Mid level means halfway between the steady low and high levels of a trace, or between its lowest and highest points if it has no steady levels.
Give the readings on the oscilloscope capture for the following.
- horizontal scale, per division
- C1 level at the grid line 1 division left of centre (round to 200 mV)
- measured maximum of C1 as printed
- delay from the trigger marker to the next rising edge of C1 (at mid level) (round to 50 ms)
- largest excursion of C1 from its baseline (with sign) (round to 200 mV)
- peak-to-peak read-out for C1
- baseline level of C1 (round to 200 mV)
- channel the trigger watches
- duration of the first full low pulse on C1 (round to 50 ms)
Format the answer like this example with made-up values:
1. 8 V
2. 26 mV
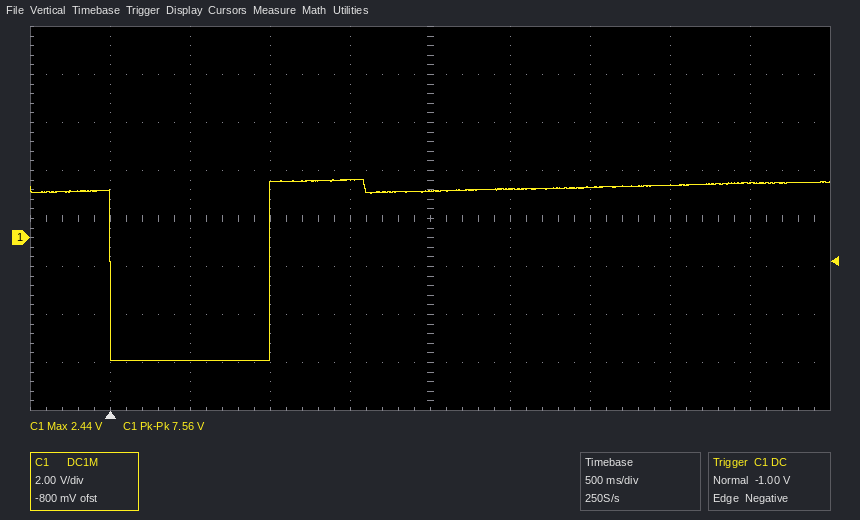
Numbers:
1. 500 ms
2. 2.4 V
3. 2.44 V
4. 1.00 s
5. -7.2 V
6. 7.56 V
7. 2.0 V
8. C1
9. 1.00 s
